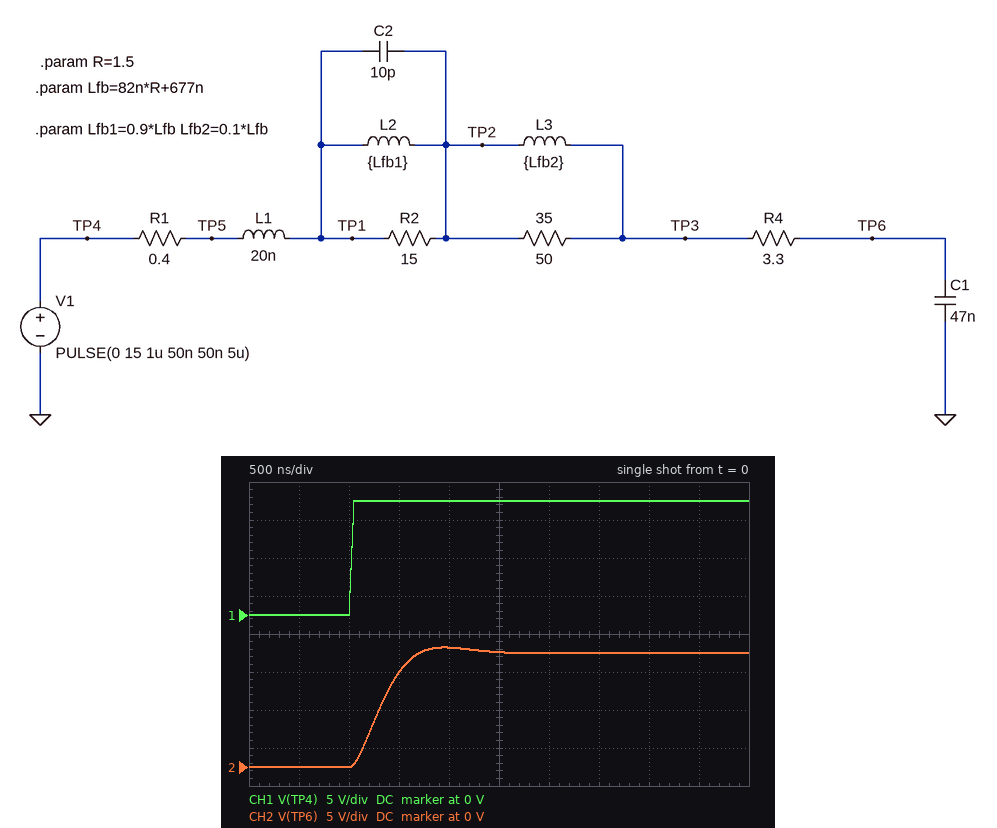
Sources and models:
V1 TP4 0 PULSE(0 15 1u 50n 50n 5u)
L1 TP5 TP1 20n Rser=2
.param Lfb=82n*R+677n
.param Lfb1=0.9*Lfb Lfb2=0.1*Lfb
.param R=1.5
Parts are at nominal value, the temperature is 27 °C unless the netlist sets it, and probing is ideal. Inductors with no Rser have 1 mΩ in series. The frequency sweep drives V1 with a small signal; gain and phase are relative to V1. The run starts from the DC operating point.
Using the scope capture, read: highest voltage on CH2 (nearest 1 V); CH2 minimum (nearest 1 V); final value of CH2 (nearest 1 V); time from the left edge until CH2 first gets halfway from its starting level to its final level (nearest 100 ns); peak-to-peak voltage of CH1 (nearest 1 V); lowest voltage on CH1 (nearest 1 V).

16 V
0 V
15 V
1.3 µs
15 V
0 V
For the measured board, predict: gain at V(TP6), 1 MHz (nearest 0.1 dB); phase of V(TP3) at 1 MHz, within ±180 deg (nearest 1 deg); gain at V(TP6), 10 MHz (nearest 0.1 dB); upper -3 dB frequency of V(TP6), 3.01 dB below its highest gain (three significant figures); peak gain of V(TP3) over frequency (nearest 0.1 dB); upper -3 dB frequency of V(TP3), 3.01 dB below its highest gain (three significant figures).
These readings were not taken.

-6.4 dB
-57 deg
-36.4 dB
738 kHz
0.3 dB
906 kHz
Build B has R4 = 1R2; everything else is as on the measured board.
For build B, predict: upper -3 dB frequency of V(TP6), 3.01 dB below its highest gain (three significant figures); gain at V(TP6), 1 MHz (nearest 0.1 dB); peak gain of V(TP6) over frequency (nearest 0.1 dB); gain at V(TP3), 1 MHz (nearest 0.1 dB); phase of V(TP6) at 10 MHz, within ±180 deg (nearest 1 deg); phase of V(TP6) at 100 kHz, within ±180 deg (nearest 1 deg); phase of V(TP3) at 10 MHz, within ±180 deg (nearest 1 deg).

883 kHz
-3.5 dB
1.4 dB
-3.0 dB
-120 deg
-6 deg
-46 deg
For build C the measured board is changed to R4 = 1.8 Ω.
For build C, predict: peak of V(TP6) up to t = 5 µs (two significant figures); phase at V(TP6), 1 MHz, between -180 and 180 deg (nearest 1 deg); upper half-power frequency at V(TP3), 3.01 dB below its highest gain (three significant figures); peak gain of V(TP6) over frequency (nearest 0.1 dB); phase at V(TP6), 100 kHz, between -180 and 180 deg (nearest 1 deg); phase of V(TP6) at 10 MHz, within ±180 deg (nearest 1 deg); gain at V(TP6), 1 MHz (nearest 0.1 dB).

17 V
-104 deg
895 kHz
0.8 dB
-7 deg
-119 deg
-4.4 dB
